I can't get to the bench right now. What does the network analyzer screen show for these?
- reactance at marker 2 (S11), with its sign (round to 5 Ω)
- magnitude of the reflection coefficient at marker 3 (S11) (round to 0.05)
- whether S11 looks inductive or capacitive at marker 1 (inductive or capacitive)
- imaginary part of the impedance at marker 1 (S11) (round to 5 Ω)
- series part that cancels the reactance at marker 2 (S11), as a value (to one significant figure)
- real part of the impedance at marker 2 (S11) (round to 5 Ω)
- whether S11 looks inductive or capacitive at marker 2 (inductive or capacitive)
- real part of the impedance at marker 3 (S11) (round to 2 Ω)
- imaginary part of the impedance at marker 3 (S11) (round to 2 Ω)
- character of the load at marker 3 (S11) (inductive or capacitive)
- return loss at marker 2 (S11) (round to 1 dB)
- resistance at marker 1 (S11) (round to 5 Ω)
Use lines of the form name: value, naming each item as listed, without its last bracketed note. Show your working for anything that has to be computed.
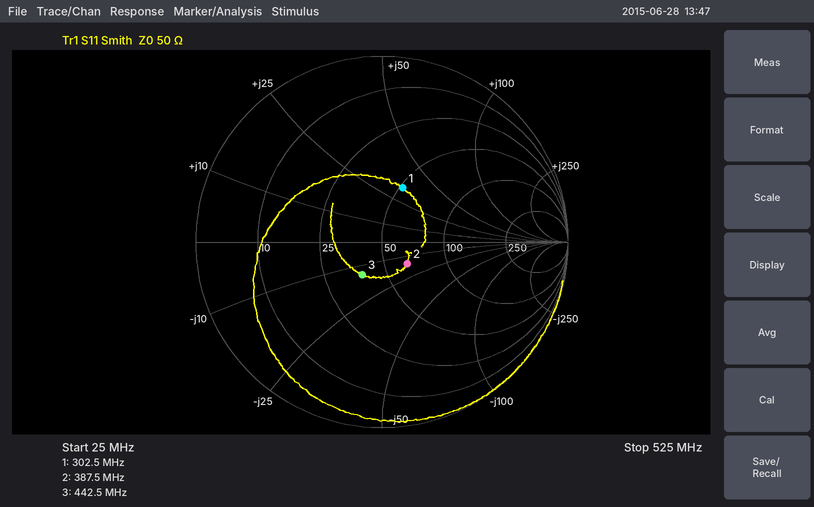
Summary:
reactance at marker 2 (S11), with its sign: -15 Ω
magnitude of the reflection coefficient at marker 3 (S11): 0.20
whether S11 looks inductive or capacitive at marker 1: inductive
imaginary part of the impedance at marker 1 (S11): +35 Ω
series part that cancels the reactance at marker 2 (S11), as a value: L = 15 Ω/(2π × 387.5 MHz) ≈ 6 nH
real part of the impedance at marker 2 (S11): 65 Ω
whether S11 looks inductive or capacitive at marker 2: capacitive
real part of the impedance at marker 3 (S11): 38 Ω
imaginary part of the impedance at marker 3 (S11): -14 Ω
character of the load at marker 3 (S11): capacitive
return loss at marker 2 (S11): 15 dB
resistance at marker 1 (S11): 50 Ω
